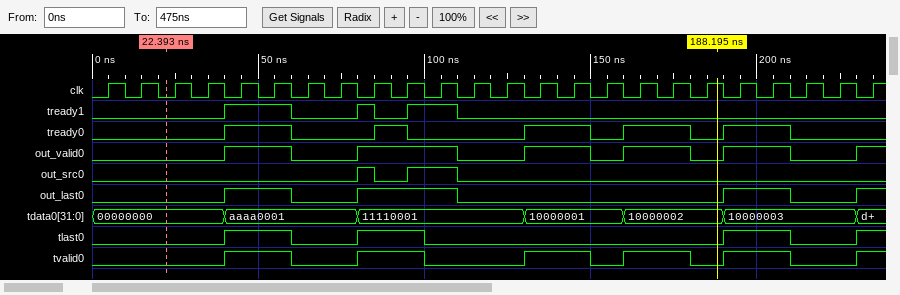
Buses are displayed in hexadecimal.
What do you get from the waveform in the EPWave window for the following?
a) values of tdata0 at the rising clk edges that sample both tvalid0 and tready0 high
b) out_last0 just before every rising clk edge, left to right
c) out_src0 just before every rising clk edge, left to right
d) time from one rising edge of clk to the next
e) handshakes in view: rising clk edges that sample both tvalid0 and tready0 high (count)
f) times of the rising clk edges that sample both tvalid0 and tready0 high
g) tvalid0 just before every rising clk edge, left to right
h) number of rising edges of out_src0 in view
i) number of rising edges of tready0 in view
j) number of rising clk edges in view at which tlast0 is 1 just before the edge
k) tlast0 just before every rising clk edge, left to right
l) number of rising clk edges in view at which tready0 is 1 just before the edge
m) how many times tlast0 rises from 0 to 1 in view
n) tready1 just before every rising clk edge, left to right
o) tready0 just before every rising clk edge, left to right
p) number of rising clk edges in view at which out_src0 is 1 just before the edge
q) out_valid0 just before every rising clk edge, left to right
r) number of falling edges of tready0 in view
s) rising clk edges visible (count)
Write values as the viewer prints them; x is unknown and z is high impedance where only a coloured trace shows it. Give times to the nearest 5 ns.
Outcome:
aaaa0001, aaaa0001, 11110001, 10000001, 10000001, 10000002, 10000002, 10000003, 10000003
0 0 0 0 1 1 0 0 1 1 1 0 0 0 0 0 0 0 0 1 1 0 0 1
0 0 0 0 0 0 0 0 1 0 1 0 0 0 0 0 0 0 0 0 0 0 0 0
10 ns
9
45 ns, 55 ns, 95 ns, 135 ns, 145 ns, 165 ns, 175 ns, 195 ns, 205 ns
0 0 0 0 1 1 0 0 1 1 0 0 0 1 1 0 1 1 0 1 1 0 0 1
2
5
7
0 0 0 0 1 1 0 0 1 1 0 0 0 0 0 0 0 0 0 1 1 0 0 1
9
4
0 0 0 0 1 1 0 0 1 0 1 0 0 0 0 0 0 0 0 0 0 0 0 0
0 0 0 0 1 1 0 0 0 1 0 0 0 1 1 0 1 1 0 1 1 0 0 0
2
0 0 0 0 1 1 0 0 1 1 1 0 0 1 1 0 1 1 0 1 1 0 0 1
5
24
